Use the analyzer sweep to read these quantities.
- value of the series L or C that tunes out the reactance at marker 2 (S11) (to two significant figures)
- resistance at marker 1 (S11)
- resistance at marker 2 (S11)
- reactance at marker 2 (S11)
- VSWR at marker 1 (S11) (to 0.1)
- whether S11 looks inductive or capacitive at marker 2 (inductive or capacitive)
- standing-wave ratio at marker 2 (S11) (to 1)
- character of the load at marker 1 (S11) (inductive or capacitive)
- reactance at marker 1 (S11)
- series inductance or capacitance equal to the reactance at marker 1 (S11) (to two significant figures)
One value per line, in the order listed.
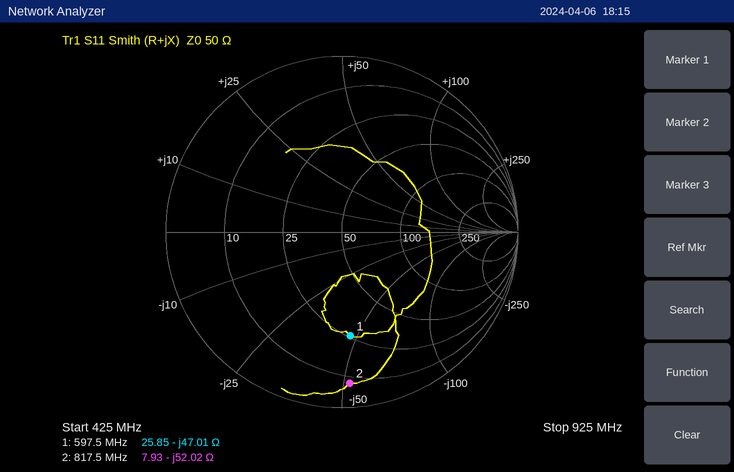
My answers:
10 nH
25.85 Ω
7.93 Ω
-52.02 Ω
3.9
capacitive
13
capacitive
-47.01 Ω
5.7 pF
